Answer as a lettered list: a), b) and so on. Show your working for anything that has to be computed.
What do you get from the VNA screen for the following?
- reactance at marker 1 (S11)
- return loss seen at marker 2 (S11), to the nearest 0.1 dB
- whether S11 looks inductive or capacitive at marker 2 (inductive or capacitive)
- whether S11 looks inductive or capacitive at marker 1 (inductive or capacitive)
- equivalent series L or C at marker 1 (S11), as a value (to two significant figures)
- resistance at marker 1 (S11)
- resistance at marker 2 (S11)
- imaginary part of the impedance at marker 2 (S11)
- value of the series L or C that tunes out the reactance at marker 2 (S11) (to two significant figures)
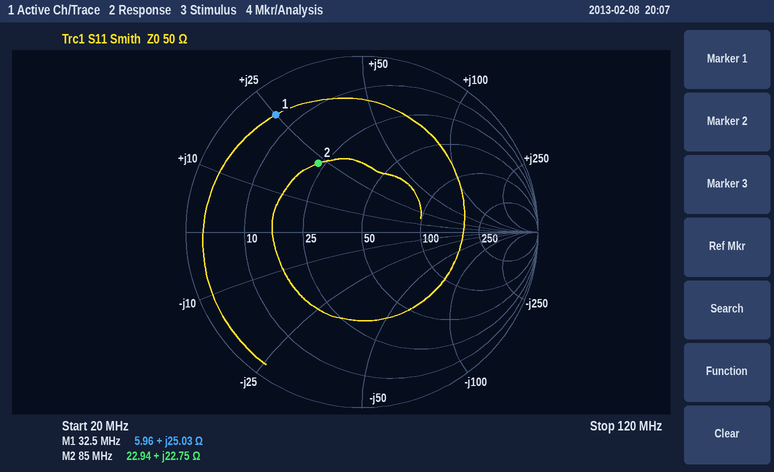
a) +25.03 Ω
b) 6.7 dB
c) inductive
d) inductive
e) L = 25.03 Ω/(2π × 32.5 MHz) ≈ 123 nH, so 120 nH to two significant figures
f) 5.96 Ω
g) 22.94 Ω
h) +22.75 Ω
i) C = 1/(2π × 85 MHz × 22.75 Ω) ≈ 82 pF
